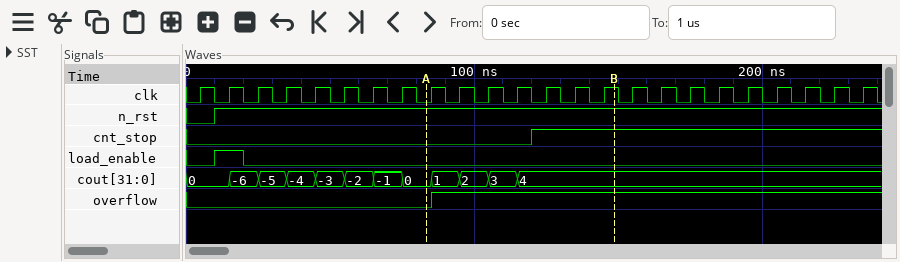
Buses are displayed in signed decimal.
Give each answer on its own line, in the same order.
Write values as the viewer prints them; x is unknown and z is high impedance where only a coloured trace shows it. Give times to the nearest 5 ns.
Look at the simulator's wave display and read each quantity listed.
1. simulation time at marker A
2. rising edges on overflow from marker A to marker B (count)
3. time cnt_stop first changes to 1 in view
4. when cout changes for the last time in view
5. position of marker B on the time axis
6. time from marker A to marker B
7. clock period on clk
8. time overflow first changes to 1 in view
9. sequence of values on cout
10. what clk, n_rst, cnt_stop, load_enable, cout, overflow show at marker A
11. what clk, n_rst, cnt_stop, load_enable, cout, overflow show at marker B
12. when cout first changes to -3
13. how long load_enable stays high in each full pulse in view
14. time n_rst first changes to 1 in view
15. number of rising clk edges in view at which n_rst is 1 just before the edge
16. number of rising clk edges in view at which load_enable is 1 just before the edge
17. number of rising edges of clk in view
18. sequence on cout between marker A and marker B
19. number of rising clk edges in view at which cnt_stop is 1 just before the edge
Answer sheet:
85 ns
1
120 ns
115 ns
150 ns
65 ns
10 ns
85 ns
0, -6, -5, -4, -3, -2, -1, 0, 1, 2, 3, 4
clk=0, n_rst=1, cnt_stop=0, load_enable=0, cout=0, overflow=0
clk=1, n_rst=1, cnt_stop=1, load_enable=0, cout=4, overflow=1
45 ns
10 ns
10 ns
23
1
24
0, 1, 2, 3, 4
12
